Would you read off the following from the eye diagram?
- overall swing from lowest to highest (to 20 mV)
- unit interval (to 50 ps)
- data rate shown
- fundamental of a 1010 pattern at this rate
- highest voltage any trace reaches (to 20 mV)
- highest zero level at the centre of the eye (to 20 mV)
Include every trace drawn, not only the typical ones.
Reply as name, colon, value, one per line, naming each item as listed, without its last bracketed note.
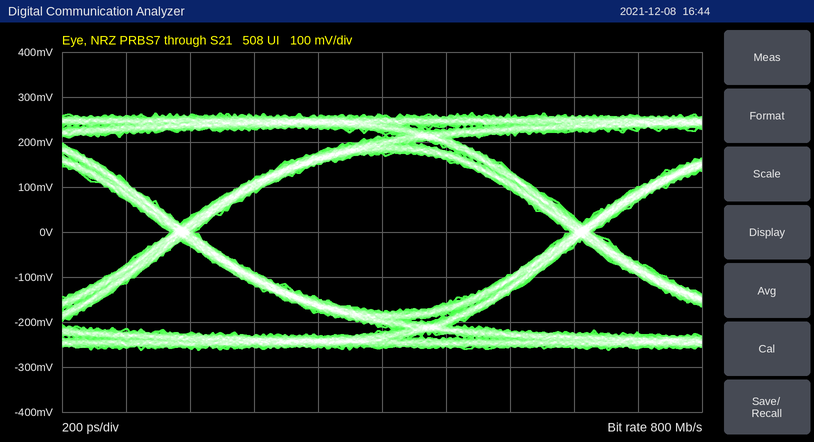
overall swing from lowest to highest: 520 mV
unit interval: 1.25 ns
data rate shown: 800 Mb/s
fundamental of a 1010 pattern at this rate: 400 MHz
highest voltage any trace reaches: 260 mV
highest zero level at the centre of the eye: -180 mV
